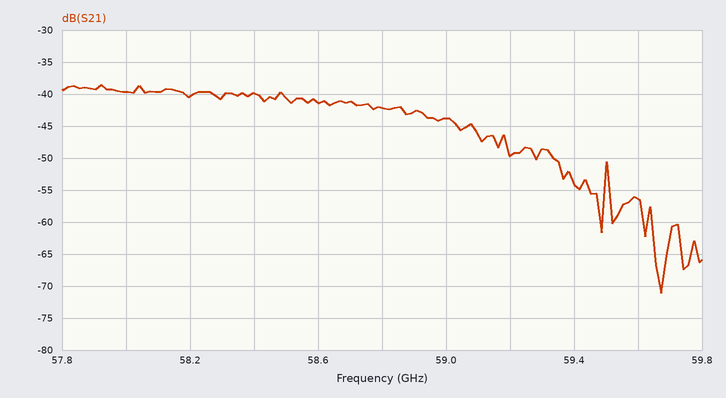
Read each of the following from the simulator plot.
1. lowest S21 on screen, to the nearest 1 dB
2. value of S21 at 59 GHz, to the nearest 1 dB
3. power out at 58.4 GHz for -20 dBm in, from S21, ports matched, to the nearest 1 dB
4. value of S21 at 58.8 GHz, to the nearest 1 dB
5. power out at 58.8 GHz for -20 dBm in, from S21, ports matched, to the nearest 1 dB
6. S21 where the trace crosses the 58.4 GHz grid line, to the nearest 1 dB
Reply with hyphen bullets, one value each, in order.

- -71 dB
- -44 dB
- -60 dBm
- -42 dB
- -62 dBm
- -40 dB
